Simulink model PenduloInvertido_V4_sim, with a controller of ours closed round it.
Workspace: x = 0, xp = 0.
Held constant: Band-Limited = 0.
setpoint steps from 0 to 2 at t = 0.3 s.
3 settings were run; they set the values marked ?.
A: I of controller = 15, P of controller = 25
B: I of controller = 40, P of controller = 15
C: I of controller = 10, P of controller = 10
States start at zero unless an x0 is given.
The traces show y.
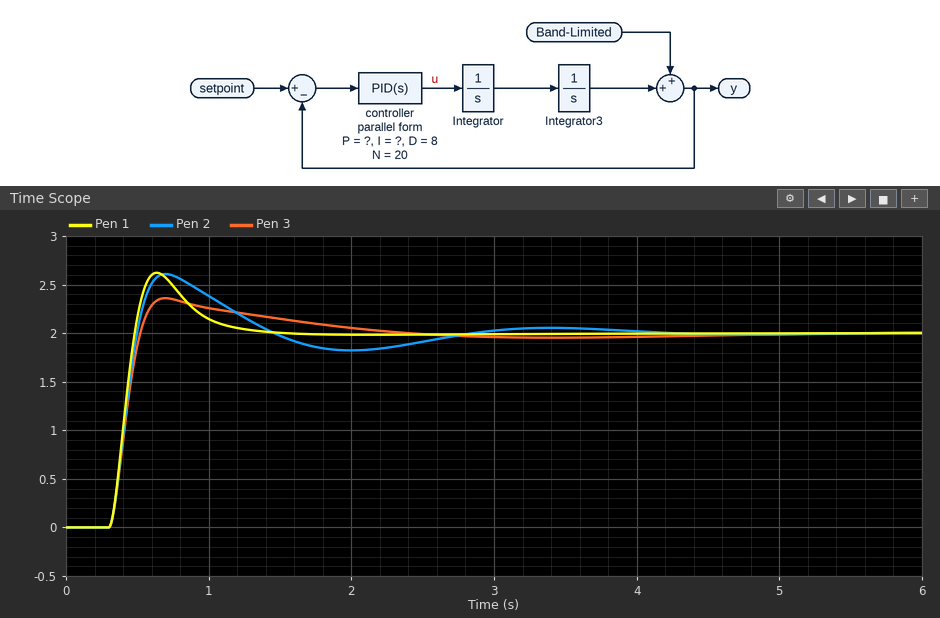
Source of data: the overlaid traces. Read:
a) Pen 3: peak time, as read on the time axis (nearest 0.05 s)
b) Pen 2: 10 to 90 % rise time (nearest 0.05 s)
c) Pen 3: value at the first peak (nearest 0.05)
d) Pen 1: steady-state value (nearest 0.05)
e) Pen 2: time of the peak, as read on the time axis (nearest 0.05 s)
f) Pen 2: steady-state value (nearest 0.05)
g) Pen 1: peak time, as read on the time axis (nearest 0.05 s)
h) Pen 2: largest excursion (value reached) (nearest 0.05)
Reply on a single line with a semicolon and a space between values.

0.70 s; 0.15 s; 2.35; 2.00; 0.70 s; 2.00; 0.65 s; 2.60
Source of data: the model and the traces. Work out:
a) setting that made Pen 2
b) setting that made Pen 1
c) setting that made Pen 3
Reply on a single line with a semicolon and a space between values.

B; A; C
